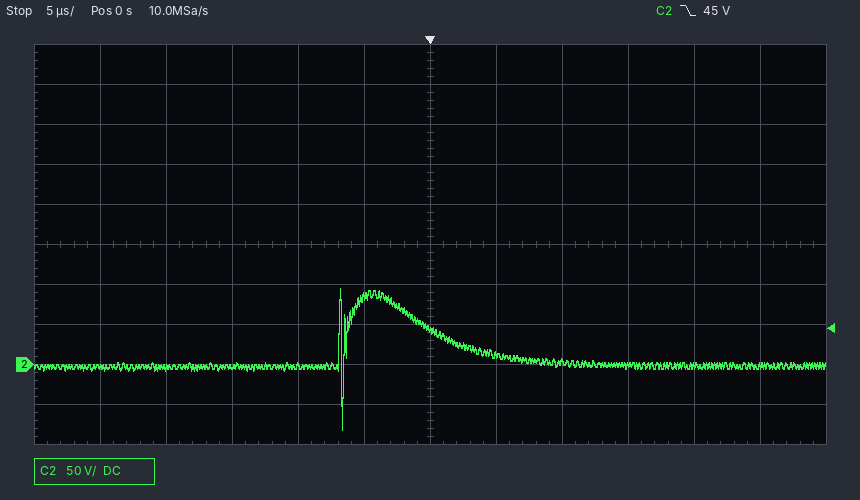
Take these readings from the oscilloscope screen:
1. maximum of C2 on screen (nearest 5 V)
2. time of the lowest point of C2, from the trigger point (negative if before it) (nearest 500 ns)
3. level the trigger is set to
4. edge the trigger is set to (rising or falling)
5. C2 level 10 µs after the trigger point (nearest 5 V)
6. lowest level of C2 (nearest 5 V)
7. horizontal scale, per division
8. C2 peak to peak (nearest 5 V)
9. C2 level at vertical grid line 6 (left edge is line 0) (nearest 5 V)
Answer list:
95 V
-6.5 µs
45 V
falling
5 V
-80 V
5 µs
175 V
45 V
